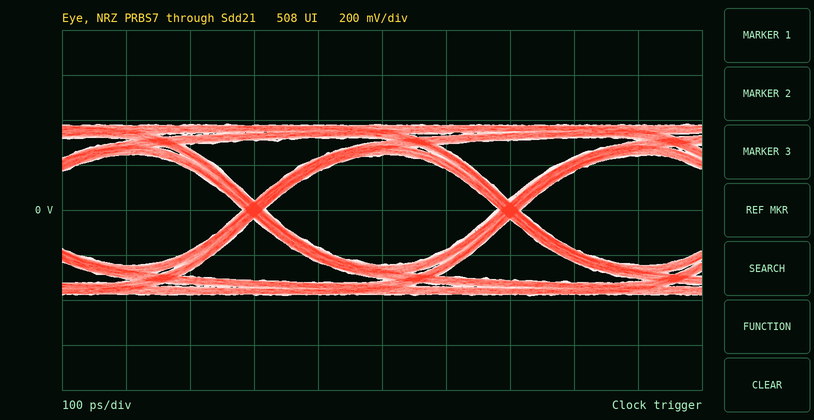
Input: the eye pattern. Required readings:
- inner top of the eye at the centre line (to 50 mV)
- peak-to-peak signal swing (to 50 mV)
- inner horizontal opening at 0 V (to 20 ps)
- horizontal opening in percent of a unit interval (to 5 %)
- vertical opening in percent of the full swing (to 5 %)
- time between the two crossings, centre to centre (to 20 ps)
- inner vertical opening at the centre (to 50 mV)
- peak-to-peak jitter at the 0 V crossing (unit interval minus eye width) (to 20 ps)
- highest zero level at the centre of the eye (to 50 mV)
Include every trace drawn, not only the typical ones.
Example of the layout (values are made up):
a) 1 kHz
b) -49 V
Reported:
a) 250 mV
b) 750 mV
c) 360 ps
d) 90 %
e) 65 %
f) 400 ps
g) 500 mV
h) 40 ps
i) -250 mV
